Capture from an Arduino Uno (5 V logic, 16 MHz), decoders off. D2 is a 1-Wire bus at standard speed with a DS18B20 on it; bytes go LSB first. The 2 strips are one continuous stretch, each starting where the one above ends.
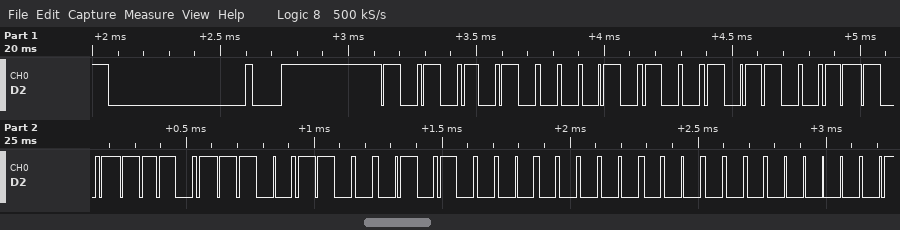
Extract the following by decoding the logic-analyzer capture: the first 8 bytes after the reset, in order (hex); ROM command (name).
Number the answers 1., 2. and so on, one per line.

1. 55 28 CD BD 33 0A 00 00
2. Match ROM
